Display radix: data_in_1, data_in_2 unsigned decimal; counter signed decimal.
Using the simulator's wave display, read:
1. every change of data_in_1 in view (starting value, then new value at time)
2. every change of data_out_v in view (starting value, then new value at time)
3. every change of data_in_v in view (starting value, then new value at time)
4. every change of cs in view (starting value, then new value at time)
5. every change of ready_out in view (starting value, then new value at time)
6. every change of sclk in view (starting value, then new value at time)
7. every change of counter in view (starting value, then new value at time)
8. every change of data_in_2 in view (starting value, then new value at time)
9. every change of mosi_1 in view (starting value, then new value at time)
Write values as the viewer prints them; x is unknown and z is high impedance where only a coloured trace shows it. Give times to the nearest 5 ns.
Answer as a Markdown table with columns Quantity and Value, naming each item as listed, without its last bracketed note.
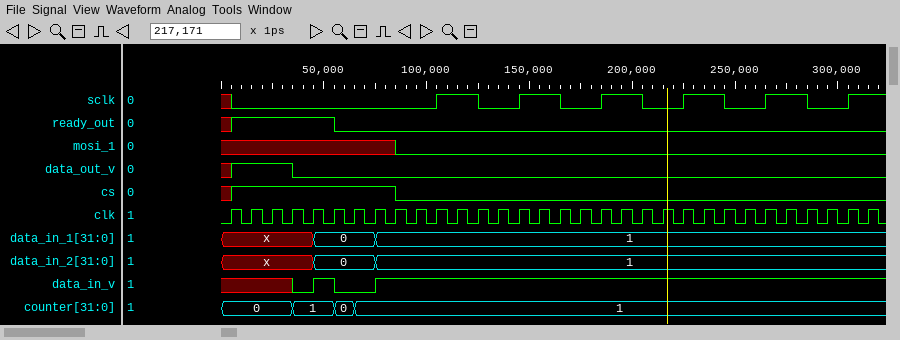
| Quantity | Value |
|---|---|
| every change of data_in_1 in view | x, 0 at 45 ns, 1 at 75 ns |
| every change of data_out_v in view | x, 1 at 5 ns, 0 at 35 ns |
| every change of data_in_v in view | x, 0 at 35 ns, 1 at 45 ns, 0 at 55 ns, 1 at 75 ns |
| every change of cs in view | x, 1 at 5 ns, 0 at 85 ns |
| every change of ready_out in view | x, 1 at 5 ns, 0 at 55 ns |
| every change of sclk in view | x, 0 at 5 ns, 1 at 105 ns, 0 at 125 ns, 1 at 145 ns, 0 at 165 ns, 1 at 185 ns, 0 at 205 ns, 1 at 225 ns, 0 at 245 ns, 1 at 265 ns, 0 at 285 ns, 1 at 305 ns |
| every change of counter in view | 0, 1 at 35 ns, 0 at 55 ns, 1 at 65 ns |
| every change of data_in_2 in view | x, 0 at 45 ns, 1 at 75 ns |
| every change of mosi_1 in view | x, 0 at 85 ns |
